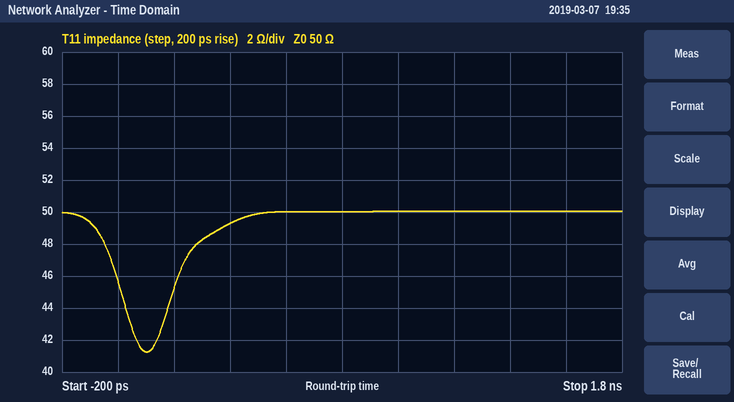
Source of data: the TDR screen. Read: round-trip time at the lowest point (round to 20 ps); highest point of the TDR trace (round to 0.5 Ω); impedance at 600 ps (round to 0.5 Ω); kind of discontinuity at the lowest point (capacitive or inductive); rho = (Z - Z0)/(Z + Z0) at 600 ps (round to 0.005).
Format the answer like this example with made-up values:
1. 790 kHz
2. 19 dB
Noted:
1. 100 ps
2. 50.0 Ω
3. 50.0 Ω
4. capacitive
5. 0.000
